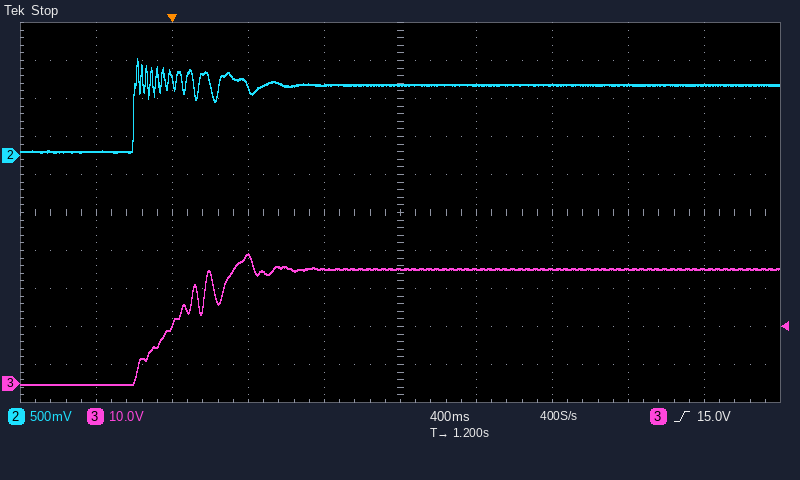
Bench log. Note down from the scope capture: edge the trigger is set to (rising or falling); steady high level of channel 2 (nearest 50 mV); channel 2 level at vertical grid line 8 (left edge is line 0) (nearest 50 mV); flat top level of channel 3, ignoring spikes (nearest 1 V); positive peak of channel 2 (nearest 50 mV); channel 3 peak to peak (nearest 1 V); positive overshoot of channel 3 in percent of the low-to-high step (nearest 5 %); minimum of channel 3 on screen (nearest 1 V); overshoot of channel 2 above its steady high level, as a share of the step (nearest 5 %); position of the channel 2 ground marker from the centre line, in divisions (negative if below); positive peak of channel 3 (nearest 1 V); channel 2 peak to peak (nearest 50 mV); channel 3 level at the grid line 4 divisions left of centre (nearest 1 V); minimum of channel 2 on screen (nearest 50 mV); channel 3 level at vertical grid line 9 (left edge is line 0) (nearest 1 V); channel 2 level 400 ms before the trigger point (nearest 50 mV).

rising
950 mV
950 mV
30 V
1.30 V
34 V
15 %
0 V
40 %
+1.5 div
34 V
1.25 V
0 V
50 mV
30 V
50 mV
